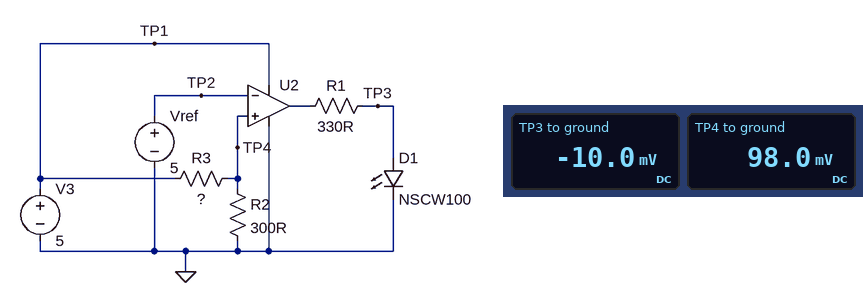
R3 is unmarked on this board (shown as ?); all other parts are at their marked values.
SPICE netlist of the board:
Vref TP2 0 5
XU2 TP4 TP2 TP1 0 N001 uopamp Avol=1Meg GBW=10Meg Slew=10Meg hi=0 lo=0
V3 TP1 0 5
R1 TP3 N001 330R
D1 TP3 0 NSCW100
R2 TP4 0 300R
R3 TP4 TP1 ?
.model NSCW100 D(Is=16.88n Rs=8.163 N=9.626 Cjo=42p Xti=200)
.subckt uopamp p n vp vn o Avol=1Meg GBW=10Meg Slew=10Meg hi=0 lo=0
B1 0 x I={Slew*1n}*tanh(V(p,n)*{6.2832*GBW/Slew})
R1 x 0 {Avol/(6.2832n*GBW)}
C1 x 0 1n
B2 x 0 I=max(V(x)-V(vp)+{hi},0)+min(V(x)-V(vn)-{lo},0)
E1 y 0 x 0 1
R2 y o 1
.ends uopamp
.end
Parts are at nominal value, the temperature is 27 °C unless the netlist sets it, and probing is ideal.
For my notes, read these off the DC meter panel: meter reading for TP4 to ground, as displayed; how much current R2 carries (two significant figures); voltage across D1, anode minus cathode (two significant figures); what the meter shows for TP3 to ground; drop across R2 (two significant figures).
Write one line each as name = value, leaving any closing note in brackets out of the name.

meter reading for TP4 to ground, as displayed = 98.0 mV
how much current R2 carries = 330 µA
voltage across D1, anode minus cathode = -10 mV
what the meter shows for TP3 to ground = -10.0 mV
drop across R2 = 98 mV
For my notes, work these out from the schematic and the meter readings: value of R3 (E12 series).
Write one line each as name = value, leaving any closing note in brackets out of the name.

value of R3 = 15 kΩ
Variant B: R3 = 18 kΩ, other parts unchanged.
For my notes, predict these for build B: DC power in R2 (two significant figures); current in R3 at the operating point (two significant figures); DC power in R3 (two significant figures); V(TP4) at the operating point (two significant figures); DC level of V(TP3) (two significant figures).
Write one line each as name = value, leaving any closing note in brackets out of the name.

DC power in R2 = 22 µW
current in R3 at the operating point = 270 µA
DC power in R3 = 1.3 mW
V(TP4) at the operating point = 82 mV
DC level of V(TP3) = -10 mV
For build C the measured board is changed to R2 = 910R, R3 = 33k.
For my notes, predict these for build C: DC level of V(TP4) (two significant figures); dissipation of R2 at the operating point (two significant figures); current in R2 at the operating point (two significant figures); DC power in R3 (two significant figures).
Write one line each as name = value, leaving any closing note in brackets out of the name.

DC level of V(TP4) = 130 mV
dissipation of R2 at the operating point = 20 µW
current in R2 at the operating point = 150 µA
DC power in R3 = 720 µW
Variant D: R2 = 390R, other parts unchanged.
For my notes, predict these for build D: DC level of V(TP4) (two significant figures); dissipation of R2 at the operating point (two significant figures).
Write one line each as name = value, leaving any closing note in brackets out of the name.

DC level of V(TP4) = 130 mV
dissipation of R2 at the operating point = 41 µW
